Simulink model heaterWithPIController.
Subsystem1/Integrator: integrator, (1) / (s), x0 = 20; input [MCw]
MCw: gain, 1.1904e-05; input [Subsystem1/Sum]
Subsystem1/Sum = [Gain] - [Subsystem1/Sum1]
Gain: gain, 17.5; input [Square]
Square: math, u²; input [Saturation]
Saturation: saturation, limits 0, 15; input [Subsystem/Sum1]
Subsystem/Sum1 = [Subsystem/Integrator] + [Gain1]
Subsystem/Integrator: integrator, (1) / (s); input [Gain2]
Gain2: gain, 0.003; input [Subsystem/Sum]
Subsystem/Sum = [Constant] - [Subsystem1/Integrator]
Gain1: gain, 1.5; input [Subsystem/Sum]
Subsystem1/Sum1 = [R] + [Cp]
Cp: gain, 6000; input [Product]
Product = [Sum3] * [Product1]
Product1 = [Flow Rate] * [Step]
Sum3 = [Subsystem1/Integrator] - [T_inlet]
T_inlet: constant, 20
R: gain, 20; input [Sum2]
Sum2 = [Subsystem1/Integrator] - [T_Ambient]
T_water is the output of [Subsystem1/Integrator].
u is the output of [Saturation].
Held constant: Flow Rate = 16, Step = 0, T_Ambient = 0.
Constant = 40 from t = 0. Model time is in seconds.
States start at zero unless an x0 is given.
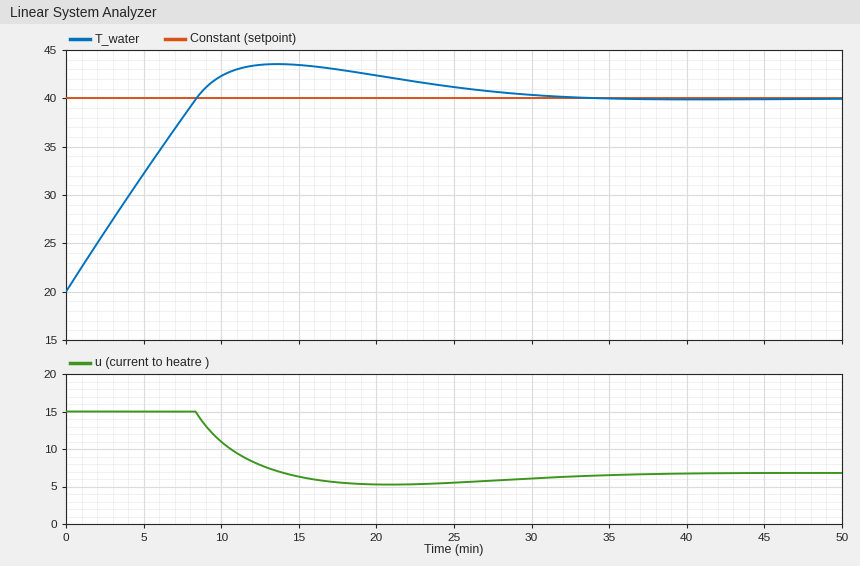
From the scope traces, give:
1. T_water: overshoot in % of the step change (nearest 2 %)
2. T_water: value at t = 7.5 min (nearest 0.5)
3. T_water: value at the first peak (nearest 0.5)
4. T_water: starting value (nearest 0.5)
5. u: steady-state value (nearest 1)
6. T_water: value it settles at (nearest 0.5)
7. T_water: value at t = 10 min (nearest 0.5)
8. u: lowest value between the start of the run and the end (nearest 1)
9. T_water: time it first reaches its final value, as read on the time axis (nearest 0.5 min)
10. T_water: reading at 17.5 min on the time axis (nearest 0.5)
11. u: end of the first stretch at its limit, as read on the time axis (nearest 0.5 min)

18 %
38.0
43.5
20.0
7
40.0
42.5
5
8.5 min
43.0
8.5 min
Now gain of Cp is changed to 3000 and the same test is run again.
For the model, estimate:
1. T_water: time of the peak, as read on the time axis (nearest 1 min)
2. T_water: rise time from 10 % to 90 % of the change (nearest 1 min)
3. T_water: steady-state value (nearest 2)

14 min
7 min
40
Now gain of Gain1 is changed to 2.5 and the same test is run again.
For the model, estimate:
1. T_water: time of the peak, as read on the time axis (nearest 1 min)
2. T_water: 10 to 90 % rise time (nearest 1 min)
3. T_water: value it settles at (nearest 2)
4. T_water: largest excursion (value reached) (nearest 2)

13 min
7 min
40
42
